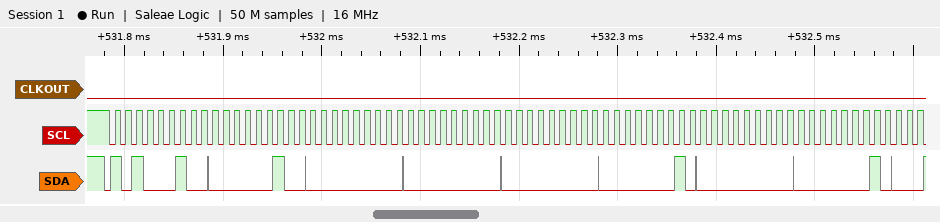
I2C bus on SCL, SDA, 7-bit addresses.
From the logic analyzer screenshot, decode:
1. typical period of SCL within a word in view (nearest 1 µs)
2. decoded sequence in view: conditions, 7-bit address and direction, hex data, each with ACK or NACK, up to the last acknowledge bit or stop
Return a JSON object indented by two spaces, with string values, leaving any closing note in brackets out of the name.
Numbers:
{
  "typical period of SCL within a word in view": "11 µs",
  "decoded sequence in view: conditions, 7-bit address and direction, hex data, each with ACK or NACK, up to the last acknowledge bit or stop": "start, address 51 write ACK, 02 ACK, 00 ACK, 00 ACK, 00 ACK, 01 ACK, 00 ACK, 01 ACK"
}
